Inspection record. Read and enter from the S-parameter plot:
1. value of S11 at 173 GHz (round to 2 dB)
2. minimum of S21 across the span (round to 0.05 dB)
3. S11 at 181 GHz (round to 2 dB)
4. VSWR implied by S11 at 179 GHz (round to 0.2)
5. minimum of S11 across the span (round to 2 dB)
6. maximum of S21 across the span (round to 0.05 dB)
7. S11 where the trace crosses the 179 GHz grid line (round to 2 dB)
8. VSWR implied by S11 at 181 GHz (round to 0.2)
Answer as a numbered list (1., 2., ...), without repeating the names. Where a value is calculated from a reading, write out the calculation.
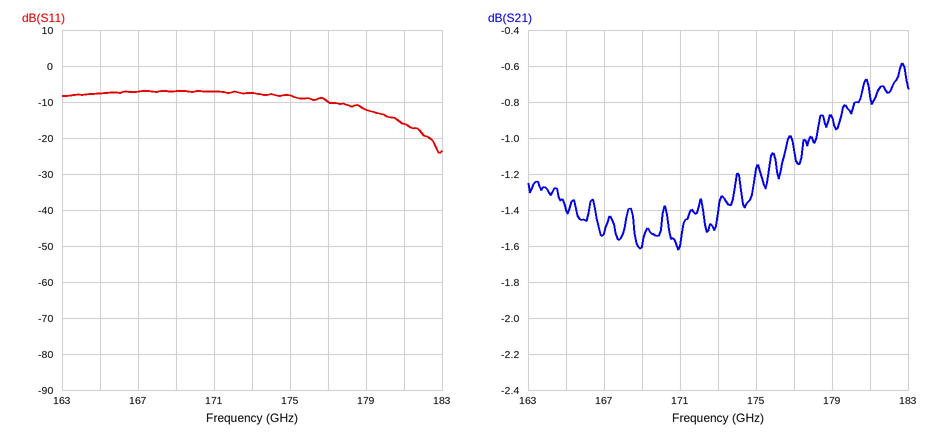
1. -8 dB
2. -1.60 dB
3. -16 dB
4. |Γ| = 10^(-12/20) = 0.2512; VSWR = (1 + 0.2512)/(1 − 0.2512) ≈ 1.67, so 1.6 to the nearest 0.2
5. -24 dB
6. -0.60 dB
7. -12 dB
8. |Γ| = 10^(-16/20) = 0.1585; VSWR = (1 + 0.1585)/(1 − 0.1585) ≈ 1.4
